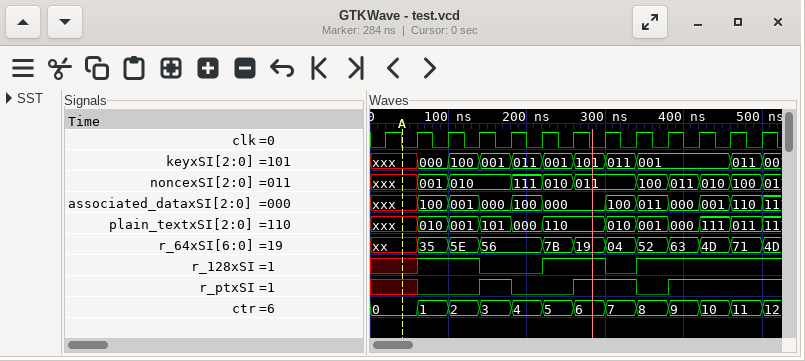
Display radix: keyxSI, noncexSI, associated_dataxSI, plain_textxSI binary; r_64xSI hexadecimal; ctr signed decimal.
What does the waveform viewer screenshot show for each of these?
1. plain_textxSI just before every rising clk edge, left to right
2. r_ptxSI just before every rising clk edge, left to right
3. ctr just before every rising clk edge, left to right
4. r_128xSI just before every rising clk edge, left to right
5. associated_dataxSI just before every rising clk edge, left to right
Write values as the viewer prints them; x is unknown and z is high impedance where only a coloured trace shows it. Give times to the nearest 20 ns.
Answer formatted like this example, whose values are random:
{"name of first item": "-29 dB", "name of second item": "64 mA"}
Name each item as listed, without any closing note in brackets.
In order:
{"plain_textxSI just before every rising clk edge, left to right": "xxx, xxx, 010, 001, 101, 000, 110, 110, 010, 001, 000, 111, 011", "r_ptxSI just before every rising clk edge, left to right": "x x 0 0 1 0 0 1 1 0 1 1 1", "ctr just before every rising clk edge, left to right": "0, 0, 1, 2, 3, 4, 5, 6, 7, 8, 9, 10, 11", "r_128xSI just before every rising clk edge, left to right": "x x 1 1 0 0 1 1 0 1 1 1 1", "associated_dataxSI just before every rising clk edge, left to right": "xxx, xxx, 100, 001, 000, 100, 000, 000, 100, 011, 000, 001, 110"}
